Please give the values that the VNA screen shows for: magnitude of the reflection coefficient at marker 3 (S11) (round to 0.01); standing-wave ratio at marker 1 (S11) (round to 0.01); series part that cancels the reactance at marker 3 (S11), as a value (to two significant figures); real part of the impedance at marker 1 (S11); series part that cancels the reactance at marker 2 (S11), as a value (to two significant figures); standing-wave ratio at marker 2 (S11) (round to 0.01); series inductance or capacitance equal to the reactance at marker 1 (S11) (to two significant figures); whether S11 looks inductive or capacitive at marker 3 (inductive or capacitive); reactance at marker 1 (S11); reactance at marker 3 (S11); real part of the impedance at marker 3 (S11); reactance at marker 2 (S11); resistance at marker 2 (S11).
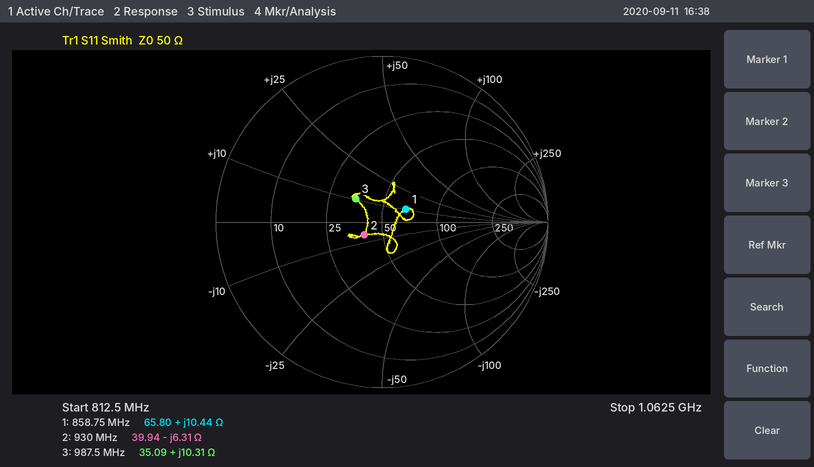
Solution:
0.21
1.39
16 pF
65.80 Ω
1.1 nH
1.30
1.9 nH
inductive
+10.44 Ω
+10.31 Ω
35.09 Ω
-6.31 Ω
39.94 Ω
